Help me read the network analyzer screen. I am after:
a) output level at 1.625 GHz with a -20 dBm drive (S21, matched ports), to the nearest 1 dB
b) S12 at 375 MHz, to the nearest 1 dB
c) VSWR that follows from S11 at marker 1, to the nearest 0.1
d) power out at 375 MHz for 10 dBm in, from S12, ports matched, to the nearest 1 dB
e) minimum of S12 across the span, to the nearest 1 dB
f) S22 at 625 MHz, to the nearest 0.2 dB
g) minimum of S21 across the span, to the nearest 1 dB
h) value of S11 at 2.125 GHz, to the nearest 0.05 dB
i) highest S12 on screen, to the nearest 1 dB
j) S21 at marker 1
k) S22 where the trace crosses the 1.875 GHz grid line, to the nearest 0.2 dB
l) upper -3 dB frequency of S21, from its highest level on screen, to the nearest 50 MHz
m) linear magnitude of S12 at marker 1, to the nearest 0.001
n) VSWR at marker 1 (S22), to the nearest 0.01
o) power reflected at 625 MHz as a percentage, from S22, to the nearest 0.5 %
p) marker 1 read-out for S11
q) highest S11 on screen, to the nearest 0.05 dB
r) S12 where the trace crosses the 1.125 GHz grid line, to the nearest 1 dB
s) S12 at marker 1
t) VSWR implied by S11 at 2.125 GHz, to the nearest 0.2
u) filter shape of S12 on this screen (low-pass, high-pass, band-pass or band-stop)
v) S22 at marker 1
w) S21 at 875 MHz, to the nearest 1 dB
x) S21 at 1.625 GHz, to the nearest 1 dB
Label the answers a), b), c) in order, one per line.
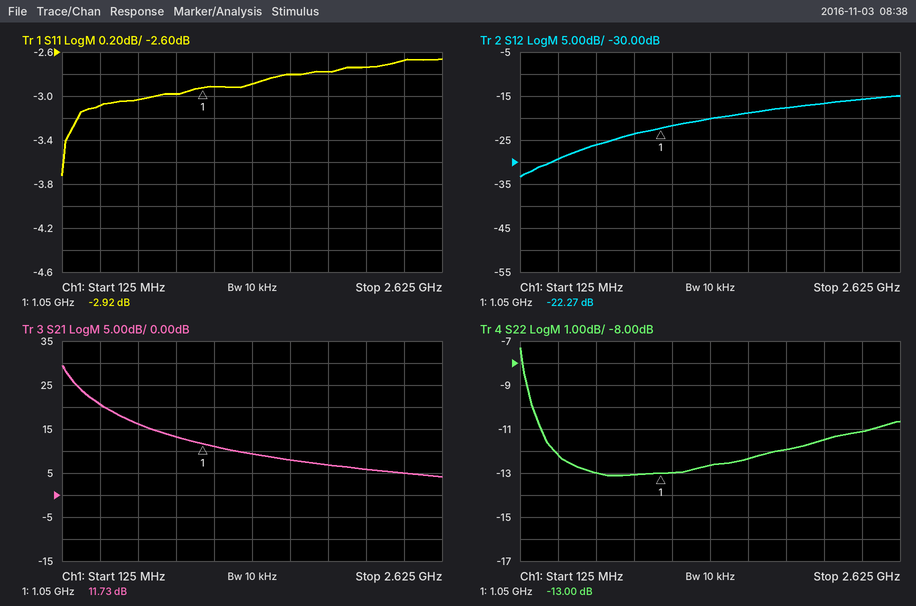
a) -12 dBm
b) -29 dB
c) 6.0
d) -19 dBm
e) -33 dB
f) -13.0 dB
g) 4 dB
h) -2.75 dB
i) -15 dB
j) 11.73 dB
k) -12.0 dB
l) 200 MHz
m) 0.077
n) 1.58
o) 5.0 %
p) -2.92 dB
q) -2.65 dB
r) -22 dB
s) -22.27 dB
t) 6.4
u) high-pass
v) -13.00 dB
w) 13 dB
x) 8 dB
